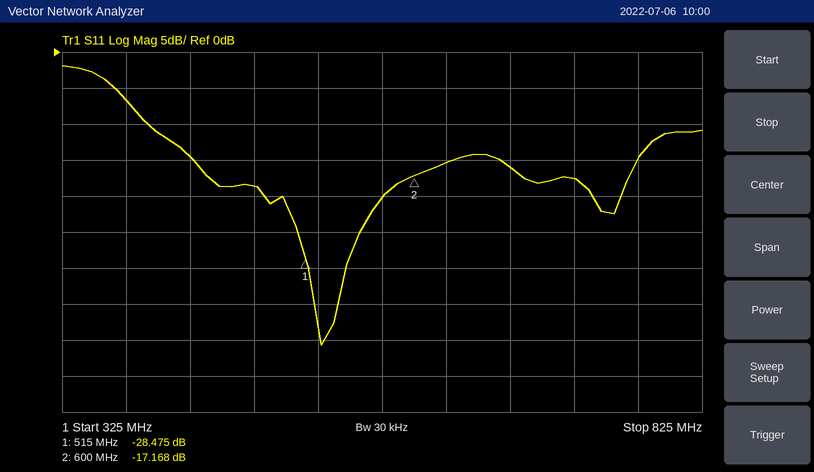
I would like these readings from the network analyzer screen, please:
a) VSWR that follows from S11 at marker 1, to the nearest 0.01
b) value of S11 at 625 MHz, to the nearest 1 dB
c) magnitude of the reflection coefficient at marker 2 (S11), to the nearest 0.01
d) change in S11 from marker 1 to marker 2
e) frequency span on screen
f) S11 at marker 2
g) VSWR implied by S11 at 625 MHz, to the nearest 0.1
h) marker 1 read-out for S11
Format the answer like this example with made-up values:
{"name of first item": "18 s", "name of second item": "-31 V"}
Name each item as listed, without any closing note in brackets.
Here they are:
{"VSWR that follows from S11 at marker 1, to the nearest 0.01": "1.08", "value of S11 at 625 MHz, to the nearest 1 dB": "-15 dB", "magnitude of the reflection coefficient at marker 2 (S11), to the nearest 0.01": "0.14", "change in S11 from marker 1 to marker 2": "11.307 dB", "frequency span on screen": "500 MHz", "S11 at marker 2": "-17.168 dB", "VSWR implied by S11 at 625 MHz, to the nearest 0.1": "1.4", "marker 1 read-out for S11": "-28.475 dB"}
